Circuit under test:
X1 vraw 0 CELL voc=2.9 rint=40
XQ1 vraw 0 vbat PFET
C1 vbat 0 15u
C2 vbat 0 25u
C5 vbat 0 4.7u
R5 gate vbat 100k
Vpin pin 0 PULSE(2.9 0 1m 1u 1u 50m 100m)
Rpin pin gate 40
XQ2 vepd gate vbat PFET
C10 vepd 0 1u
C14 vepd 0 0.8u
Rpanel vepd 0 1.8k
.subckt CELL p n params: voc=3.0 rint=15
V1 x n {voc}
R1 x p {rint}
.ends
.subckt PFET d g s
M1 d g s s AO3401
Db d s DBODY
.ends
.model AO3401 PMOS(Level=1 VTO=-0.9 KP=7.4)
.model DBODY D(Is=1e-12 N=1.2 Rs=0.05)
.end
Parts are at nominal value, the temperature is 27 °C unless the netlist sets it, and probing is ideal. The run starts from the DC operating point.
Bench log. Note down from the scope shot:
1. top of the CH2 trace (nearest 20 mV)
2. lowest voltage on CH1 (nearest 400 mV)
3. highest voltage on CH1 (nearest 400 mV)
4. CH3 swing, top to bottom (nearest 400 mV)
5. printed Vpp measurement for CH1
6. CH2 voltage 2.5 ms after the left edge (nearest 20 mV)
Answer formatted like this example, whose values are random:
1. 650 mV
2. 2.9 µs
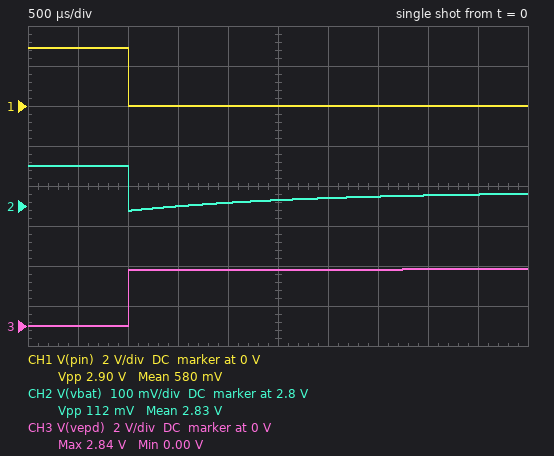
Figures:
1. 2.90 V
2. 0 V
3. 2.8 V
4. 2.8 V
5. 2.90 V
6. 2.82 V
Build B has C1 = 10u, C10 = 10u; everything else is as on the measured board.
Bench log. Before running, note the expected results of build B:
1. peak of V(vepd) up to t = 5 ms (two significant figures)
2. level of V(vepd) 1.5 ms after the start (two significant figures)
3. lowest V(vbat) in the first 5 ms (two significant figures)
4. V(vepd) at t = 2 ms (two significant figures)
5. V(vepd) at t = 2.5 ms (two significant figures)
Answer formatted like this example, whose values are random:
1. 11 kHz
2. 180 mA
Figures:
1. 2.8 V
2. 2.4 V
3. 2.3 V
4. 2.5 V
5. 2.6 V
